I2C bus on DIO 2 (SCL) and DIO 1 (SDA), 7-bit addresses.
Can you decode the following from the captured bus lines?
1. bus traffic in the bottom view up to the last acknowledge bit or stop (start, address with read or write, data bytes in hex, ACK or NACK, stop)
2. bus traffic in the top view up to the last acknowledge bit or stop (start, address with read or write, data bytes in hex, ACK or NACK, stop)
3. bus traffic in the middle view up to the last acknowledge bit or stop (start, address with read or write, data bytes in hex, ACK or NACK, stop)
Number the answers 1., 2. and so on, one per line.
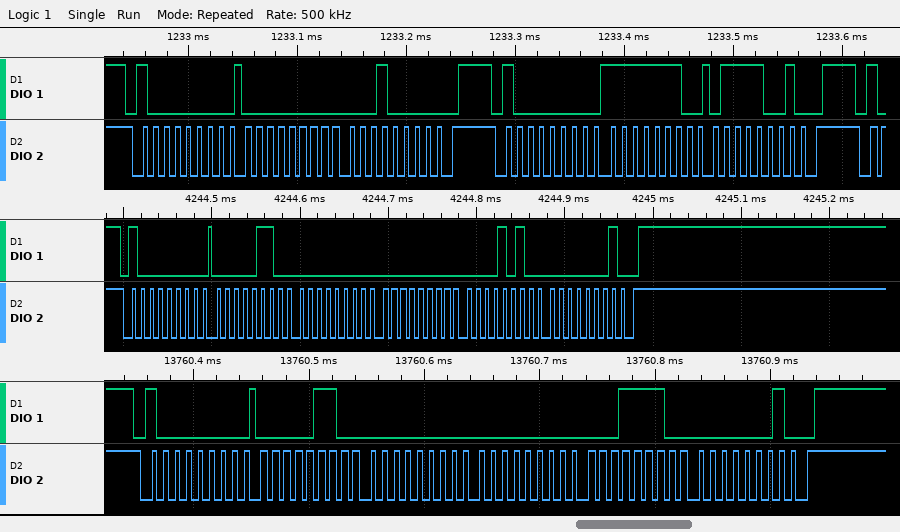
1. start, address 40 write ACK, 06 ACK, 00 ACK, 00 ACK, 1E ACK, 01 ACK, stop
2. start, address 40 write ACK, 00 ACK, 10 ACK, stop, start, address 40 write ACK, FE ACK, 79 ACK, stop
3. start, address 40 write ACK, 06 ACK, 00 ACK, 00 ACK, 0A ACK, 01 ACK, stop
